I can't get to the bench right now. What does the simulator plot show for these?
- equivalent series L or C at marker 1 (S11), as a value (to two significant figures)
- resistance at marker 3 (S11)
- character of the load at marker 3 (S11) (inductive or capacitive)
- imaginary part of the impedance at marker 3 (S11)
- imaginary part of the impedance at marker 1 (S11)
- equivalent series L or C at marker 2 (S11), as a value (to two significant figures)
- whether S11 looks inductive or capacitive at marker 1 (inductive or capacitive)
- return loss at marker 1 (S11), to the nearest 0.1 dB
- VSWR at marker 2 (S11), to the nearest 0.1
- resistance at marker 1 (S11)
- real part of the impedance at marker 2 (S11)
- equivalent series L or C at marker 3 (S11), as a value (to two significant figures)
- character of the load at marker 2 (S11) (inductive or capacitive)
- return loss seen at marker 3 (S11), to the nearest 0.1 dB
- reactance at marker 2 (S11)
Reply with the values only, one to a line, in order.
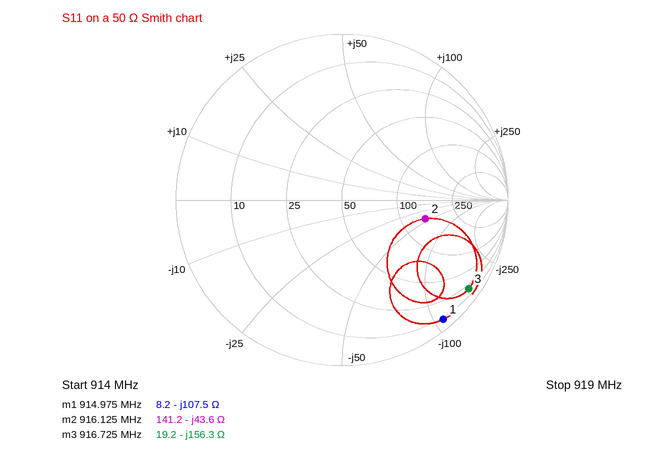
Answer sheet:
1.6 pF
19.2 Ω
capacitive
-156.3 Ω
-107.5 Ω
4.0 pF
capacitive
0.5 dB
3.1
8.2 Ω
141.2 Ω
1.1 pF
capacitive
0.6 dB
-43.6 Ω
